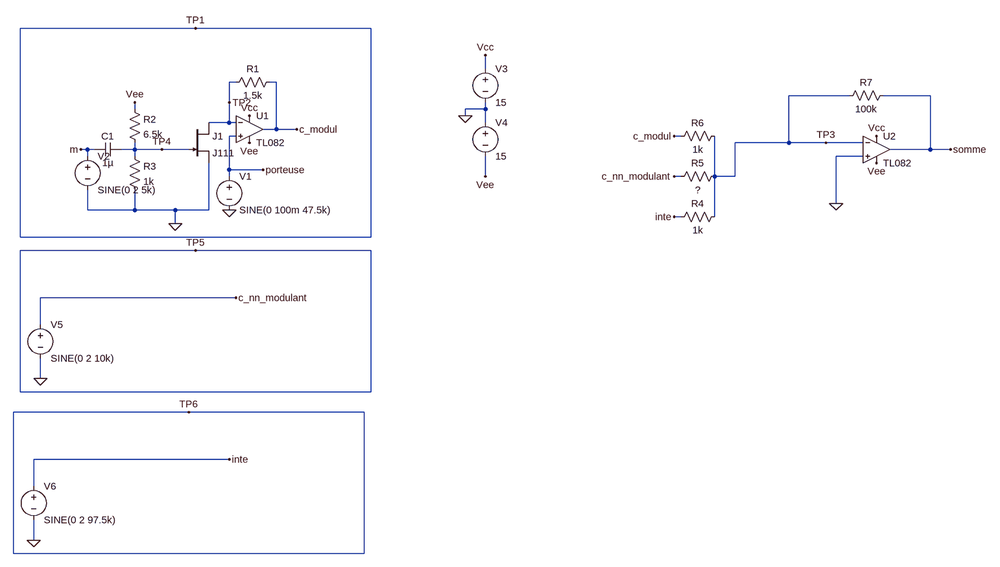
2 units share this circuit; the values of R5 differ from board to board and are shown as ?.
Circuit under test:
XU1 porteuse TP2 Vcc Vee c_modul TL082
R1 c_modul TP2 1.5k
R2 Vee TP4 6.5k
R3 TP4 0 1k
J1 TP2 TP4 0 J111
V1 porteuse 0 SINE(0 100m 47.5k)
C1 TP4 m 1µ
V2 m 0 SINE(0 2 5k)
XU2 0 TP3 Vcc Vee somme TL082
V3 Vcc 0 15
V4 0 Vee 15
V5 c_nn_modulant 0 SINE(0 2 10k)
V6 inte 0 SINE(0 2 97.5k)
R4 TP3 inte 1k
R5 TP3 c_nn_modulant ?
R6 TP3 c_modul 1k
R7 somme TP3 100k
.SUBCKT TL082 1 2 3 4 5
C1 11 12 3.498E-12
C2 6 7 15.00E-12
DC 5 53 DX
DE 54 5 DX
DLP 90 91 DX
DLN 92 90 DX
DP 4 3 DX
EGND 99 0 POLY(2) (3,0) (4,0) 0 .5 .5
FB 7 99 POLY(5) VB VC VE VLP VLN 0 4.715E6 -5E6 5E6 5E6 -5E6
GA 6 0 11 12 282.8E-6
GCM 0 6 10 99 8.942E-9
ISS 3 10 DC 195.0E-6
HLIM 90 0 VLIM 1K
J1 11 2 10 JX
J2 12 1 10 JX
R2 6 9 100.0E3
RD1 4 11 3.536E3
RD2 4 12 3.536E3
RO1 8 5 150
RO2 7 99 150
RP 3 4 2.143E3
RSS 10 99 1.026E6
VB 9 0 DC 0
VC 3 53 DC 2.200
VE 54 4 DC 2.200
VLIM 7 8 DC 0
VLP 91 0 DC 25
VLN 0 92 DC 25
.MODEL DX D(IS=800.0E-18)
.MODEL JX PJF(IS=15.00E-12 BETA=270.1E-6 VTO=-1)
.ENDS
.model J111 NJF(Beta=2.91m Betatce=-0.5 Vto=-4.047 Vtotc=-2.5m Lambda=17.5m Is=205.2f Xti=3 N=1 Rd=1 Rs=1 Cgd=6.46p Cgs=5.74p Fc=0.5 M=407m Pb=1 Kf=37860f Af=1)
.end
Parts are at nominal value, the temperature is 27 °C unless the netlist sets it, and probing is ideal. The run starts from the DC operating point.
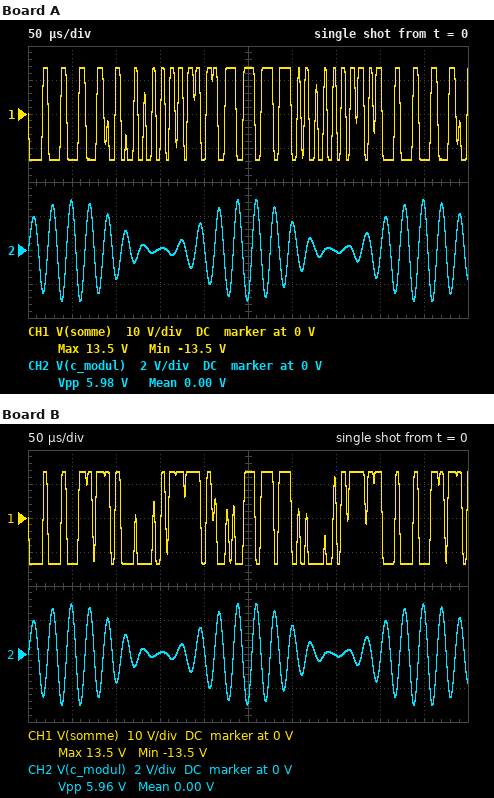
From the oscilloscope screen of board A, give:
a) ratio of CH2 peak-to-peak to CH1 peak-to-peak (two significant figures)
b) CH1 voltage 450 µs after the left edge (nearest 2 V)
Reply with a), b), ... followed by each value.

a) 0.22
b) -14 V
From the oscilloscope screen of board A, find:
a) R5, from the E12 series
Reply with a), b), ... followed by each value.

a) 3.3 kΩ
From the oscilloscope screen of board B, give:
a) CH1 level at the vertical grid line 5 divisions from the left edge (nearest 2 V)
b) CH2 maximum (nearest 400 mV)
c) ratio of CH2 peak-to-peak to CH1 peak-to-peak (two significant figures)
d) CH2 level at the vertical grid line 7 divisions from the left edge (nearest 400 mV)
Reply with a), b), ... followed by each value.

a) 14 V
b) 2.8 V
c) 0.22
d) 0 V
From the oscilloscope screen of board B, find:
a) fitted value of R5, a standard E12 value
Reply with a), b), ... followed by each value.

a) 1.2 kΩ
